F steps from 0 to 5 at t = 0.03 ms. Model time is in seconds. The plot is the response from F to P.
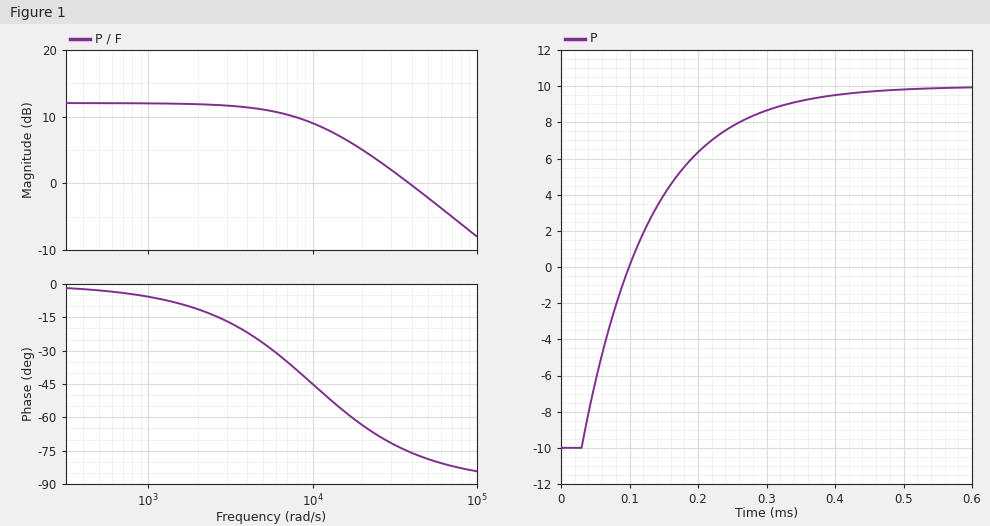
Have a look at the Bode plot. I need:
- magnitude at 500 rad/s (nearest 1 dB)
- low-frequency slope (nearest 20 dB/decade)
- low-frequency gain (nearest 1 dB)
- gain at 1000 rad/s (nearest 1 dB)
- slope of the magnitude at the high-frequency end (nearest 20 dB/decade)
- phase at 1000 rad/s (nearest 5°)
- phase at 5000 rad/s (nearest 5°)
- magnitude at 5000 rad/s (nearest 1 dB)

12 dB
0 dB/decade
12 dB
12 dB
-20 dB/decade
-5°
-25°
11 dB
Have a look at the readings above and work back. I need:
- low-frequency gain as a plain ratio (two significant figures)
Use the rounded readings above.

4.0
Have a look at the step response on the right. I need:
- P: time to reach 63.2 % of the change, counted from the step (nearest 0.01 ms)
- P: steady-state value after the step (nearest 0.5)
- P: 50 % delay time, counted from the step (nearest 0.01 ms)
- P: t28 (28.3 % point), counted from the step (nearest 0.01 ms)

0.10 ms
10.0
0.07 ms
0.03 ms
